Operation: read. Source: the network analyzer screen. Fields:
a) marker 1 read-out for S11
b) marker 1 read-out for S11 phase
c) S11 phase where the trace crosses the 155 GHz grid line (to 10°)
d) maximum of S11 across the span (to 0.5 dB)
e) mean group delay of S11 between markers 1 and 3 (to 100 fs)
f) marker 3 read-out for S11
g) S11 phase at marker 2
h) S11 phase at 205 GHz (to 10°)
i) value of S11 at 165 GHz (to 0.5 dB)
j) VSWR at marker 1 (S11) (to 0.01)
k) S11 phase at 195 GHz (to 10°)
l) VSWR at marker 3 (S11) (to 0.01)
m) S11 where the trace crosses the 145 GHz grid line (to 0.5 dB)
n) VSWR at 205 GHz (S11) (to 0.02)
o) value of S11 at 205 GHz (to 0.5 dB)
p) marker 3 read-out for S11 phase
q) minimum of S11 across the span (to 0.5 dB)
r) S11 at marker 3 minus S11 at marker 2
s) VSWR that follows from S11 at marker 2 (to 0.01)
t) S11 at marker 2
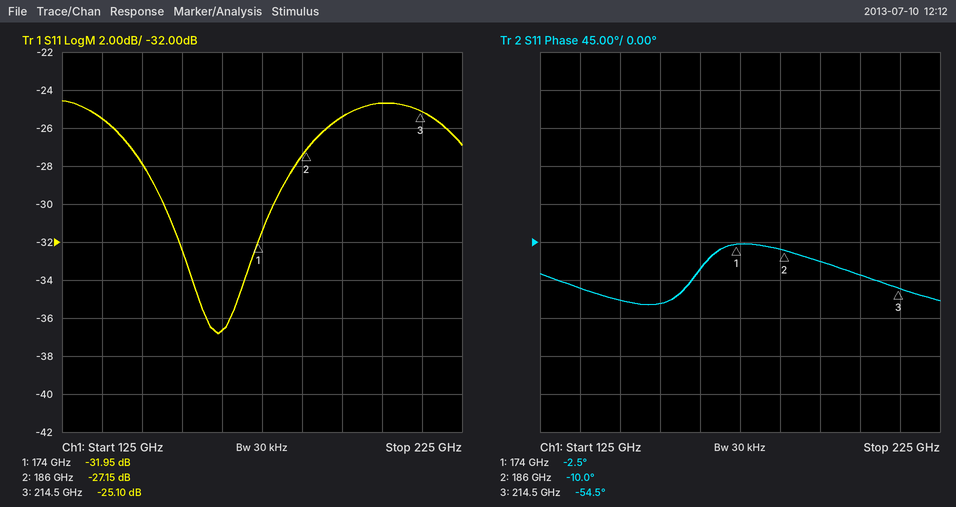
-31.95 dB
-2.5°
-70°
-24.5 dB
3.6 ps
-25.10 dB
-10.0°
-40°
-36.5 dB
1.05
-20°
1.12
-28.0 dB
1.12
-24.5 dB
-54.5°
-37.0 dB
2.05 dB
1.09
-27.15 dB
